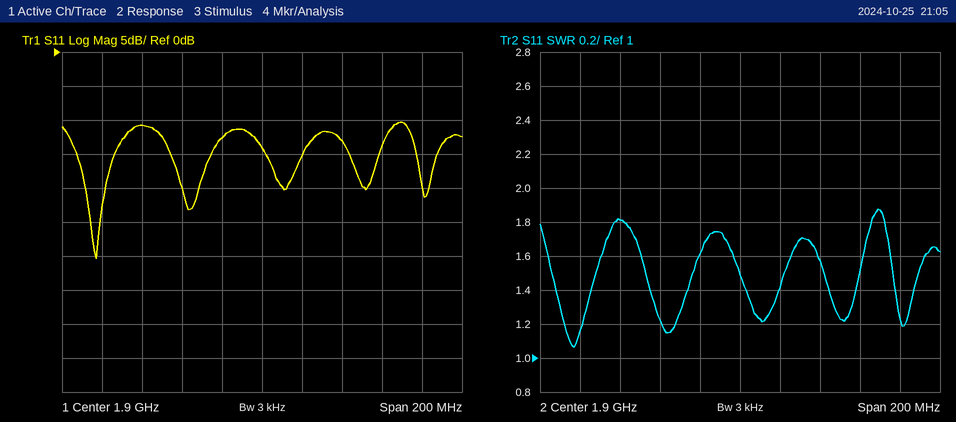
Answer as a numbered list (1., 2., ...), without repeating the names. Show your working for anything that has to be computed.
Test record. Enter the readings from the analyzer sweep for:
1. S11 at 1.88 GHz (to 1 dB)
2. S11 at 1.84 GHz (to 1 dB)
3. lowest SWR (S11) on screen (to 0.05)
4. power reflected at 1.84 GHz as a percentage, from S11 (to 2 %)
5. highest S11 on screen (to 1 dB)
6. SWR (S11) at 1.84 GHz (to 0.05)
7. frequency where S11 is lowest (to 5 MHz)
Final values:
1. -13 dB
2. -11 dB
3. 1.05
4. 10^(-11/10) ≈ 8 %
5. -10 dB
6. 1.80
7. 1.815 GHz
